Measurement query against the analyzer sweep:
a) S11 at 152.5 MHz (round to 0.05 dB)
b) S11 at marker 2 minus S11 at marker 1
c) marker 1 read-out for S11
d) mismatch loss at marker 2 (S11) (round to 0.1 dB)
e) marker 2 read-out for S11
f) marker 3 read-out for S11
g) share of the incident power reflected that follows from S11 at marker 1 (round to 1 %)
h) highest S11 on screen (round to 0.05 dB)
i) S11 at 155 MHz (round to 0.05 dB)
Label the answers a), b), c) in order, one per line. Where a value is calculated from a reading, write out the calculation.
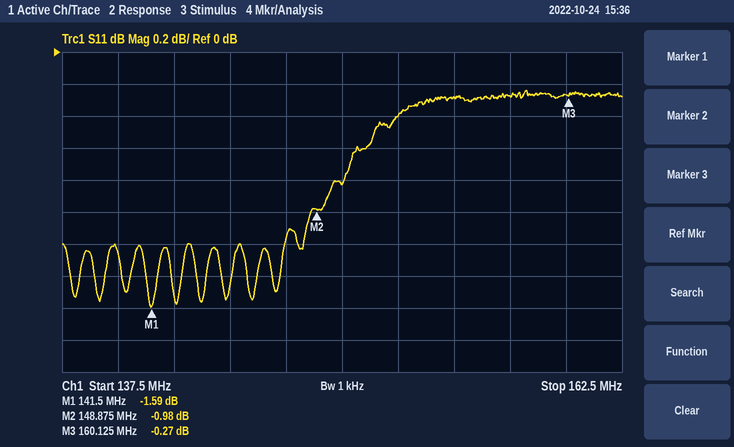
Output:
a) -0.40 dB
b) -0.98 − (-1.59) = 0.61 dB
c) -1.59 dB
d) −10 log10(1 − 10^(-0.98/10)) ≈ 6.9 dB
e) -0.98 dB
f) -0.27 dB
g) 10^(-1.59/10) ≈ 69 %
h) -0.25 dB
i) -0.30 dB
